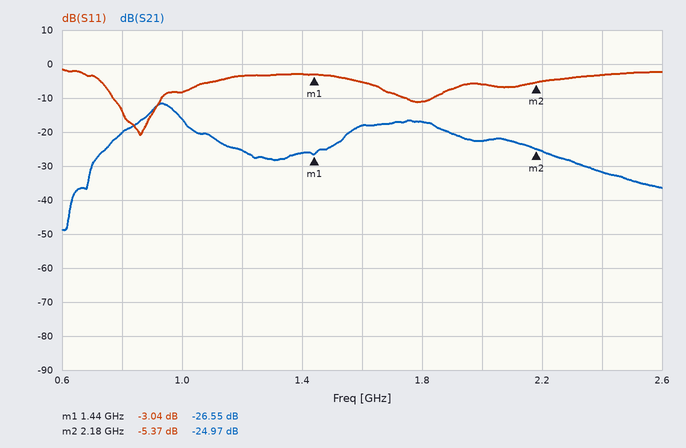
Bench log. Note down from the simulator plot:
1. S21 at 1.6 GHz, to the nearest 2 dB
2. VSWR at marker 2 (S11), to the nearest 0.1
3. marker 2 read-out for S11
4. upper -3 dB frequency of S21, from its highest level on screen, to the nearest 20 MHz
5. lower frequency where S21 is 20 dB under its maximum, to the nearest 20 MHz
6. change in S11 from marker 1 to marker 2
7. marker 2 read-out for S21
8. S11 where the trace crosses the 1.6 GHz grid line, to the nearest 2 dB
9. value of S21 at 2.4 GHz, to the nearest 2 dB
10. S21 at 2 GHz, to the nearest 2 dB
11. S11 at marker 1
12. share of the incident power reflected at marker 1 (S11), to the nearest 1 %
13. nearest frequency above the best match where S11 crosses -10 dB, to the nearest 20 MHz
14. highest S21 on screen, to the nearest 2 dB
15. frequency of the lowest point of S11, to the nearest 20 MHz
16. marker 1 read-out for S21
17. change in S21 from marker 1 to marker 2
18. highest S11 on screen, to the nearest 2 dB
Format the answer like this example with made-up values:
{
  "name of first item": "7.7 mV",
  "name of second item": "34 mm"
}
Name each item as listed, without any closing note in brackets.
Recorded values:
{
  "S21 at 1.6 GHz, to the nearest 2 dB": "-18 dB",
  "VSWR at marker 2 (S11), to the nearest 0.1": "3.3",
  "marker 2 read-out for S11": "-5.37 dB",
  "upper -3 dB frequency of S21, from its highest level on screen, to the nearest 20 MHz": "980 MHz",
  "lower frequency where S21 is 20 dB under its maximum, to the nearest 20 MHz": "700 MHz",
  "change in S11 from marker 1 to marker 2": "-2.33 dB",
  "marker 2 read-out for S21": "-24.97 dB",
  "S11 where the trace crosses the 1.6 GHz grid line, to the nearest 2 dB": "-6 dB",
  "value of S21 at 2.4 GHz, to the nearest 2 dB": "-32 dB",
  "S21 at 2 GHz, to the nearest 2 dB": "-22 dB",
  "S11 at marker 1": "-3.04 dB",
  "share of the incident power reflected at marker 1 (S11), to the nearest 1 %": "50 %",
  "nearest frequency above the best match where S11 crosses -10 dB, to the nearest 20 MHz": "940 MHz",
  "highest S21 on screen, to the nearest 2 dB": "-12 dB",
  "frequency of the lowest point of S11, to the nearest 20 MHz": "860 MHz",
  "marker 1 read-out for S21": "-26.55 dB",
  "change in S21 from marker 1 to marker 2": "1.58 dB",
  "highest S11 on screen, to the nearest 2 dB": "-2 dB"
}
